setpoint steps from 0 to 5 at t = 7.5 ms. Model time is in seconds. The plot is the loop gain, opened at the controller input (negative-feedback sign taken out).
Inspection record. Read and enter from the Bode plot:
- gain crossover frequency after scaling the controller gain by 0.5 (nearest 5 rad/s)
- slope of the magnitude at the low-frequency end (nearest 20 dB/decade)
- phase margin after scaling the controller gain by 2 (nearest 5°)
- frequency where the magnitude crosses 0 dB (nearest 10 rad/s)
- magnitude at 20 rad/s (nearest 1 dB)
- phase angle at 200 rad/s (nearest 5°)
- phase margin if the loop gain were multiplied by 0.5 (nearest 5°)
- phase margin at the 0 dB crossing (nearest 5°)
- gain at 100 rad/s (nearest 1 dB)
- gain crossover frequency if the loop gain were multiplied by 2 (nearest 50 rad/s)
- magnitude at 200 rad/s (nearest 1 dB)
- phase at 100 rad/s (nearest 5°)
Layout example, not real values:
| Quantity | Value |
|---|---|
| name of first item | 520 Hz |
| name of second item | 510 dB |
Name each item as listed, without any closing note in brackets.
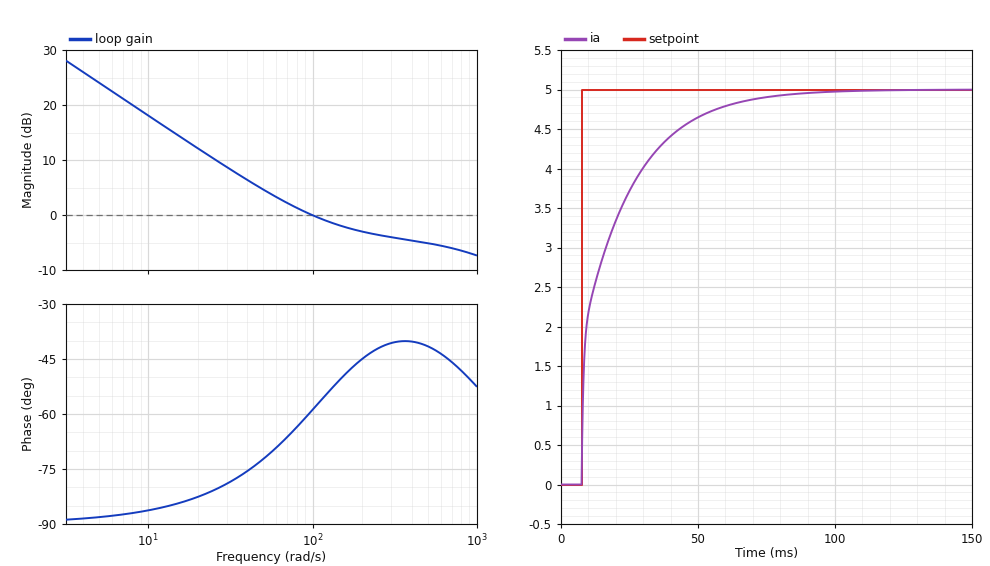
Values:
| Quantity | Value |
|---|---|
| gain crossover frequency after scaling the controller gain by 0.5 | 40 rad/s |
| slope of the magnitude at the low-frequency end | -20 dB/decade |
| phase margin after scaling the controller gain by 2 | 135° |
| frequency where the magnitude crosses 0 dB | 100 rad/s |
| magnitude at 20 rad/s | 12 dB |
| phase angle at 200 rad/s | -45° |
| phase margin if the loop gain were multiplied by 0.5 | 105° |
| phase margin at the 0 dB crossing | 120° |
| gain at 100 rad/s | 0 dB |
| gain crossover frequency if the loop gain were multiplied by 2 | 700 rad/s |
| magnitude at 200 rad/s | -3 dB |
| phase at 100 rad/s | -60° |
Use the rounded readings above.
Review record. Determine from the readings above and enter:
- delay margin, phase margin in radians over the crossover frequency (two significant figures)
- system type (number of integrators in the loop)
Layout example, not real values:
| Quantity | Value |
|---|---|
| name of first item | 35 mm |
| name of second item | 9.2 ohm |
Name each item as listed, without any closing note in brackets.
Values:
| Quantity | Value |
|---|---|
| delay margin, phase margin in radians over the crossover frequency | 0.021 s |
| system type | 1 |
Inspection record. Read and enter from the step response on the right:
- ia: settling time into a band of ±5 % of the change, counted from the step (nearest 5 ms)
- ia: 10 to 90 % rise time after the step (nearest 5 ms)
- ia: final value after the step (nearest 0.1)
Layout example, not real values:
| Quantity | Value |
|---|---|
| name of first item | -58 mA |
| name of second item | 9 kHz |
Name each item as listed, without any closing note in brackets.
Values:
| Quantity | Value |
|---|---|
| ia: settling time into a band of ±5 % of the change, counted from the step | 50 ms |
| ia: 10 to 90 % rise time after the step | 35 ms |
| ia: final value after the step | 5.0 |
